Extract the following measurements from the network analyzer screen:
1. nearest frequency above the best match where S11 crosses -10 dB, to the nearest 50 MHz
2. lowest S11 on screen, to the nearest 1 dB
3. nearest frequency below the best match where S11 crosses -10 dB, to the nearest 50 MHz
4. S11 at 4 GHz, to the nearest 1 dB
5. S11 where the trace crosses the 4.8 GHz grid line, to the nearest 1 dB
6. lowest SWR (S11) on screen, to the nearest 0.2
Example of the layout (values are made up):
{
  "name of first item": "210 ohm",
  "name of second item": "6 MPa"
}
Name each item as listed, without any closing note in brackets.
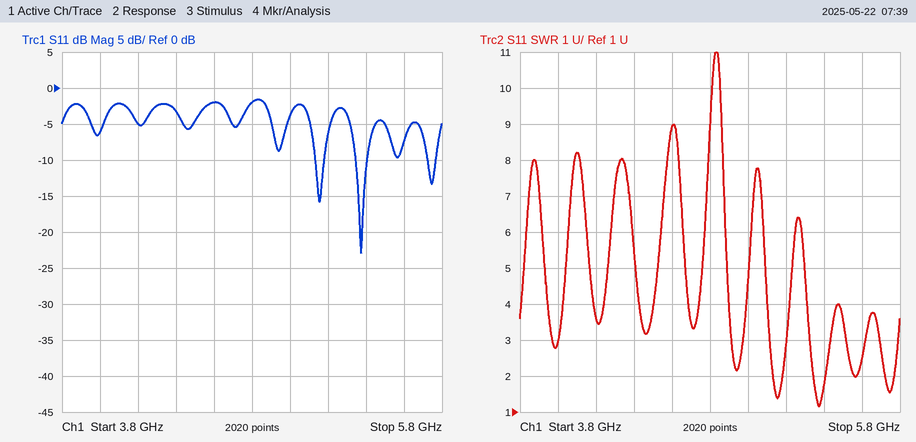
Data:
{
  "nearest frequency above the best match where S11 crosses -10 dB, to the nearest 50 MHz": "5.40 GHz",
  "lowest S11 on screen, to the nearest 1 dB": "-23 dB",
  "nearest frequency below the best match where S11 crosses -10 dB, to the nearest 50 MHz": "5.35 GHz",
  "S11 at 4 GHz, to the nearest 1 dB": "-6 dB",
  "S11 where the trace crosses the 4.8 GHz grid line, to the nearest 1 dB": "-2 dB",
  "lowest SWR (S11) on screen, to the nearest 0.2": "1.2"
}
